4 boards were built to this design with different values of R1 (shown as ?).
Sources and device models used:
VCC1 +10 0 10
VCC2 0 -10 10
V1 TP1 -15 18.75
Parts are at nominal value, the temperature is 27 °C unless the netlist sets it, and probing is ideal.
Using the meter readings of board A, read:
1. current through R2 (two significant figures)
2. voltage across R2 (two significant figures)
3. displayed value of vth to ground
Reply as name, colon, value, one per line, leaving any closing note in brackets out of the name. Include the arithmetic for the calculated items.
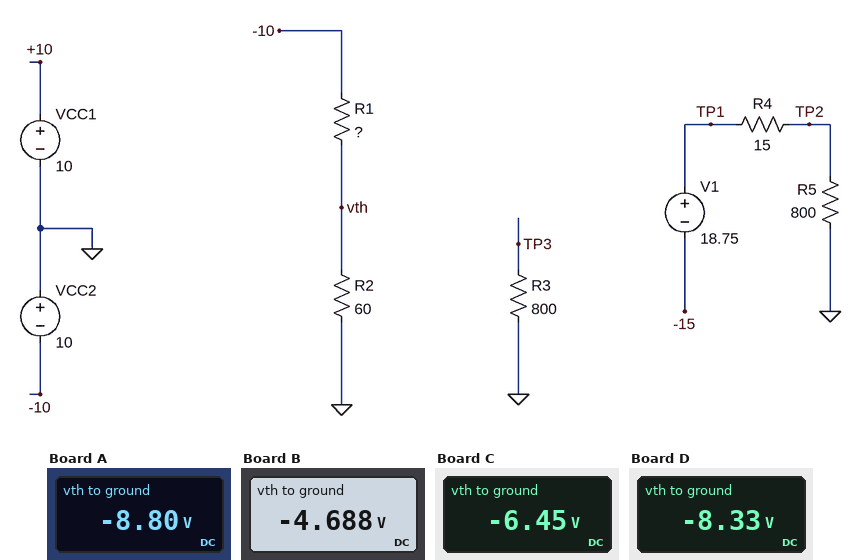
current through R2: (0 V - (-8.8 V)) / 60 Ω = 150 mA
voltage across R2: 0 V - (-8.8 V) = 8.8 V
displayed value of vth to ground: -8.80 V
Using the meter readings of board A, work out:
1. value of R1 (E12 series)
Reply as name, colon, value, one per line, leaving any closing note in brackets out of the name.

value of R1: 8.2 Ω
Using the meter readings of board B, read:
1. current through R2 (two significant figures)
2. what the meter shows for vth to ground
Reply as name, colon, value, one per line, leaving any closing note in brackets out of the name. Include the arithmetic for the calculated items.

current through R2: (0 V - (-4.688 V)) / 60 Ω = 78 mA
what the meter shows for vth to ground: -4.688 V
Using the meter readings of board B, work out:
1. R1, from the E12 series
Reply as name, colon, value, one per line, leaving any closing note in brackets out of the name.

R1, from the E12 series: 68 Ω
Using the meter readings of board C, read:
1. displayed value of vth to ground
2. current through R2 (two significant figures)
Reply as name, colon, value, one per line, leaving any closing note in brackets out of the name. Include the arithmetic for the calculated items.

displayed value of vth to ground: -6.45 V
current through R2: (0 V - (-6.45 V)) / 60 Ω = 110 mA
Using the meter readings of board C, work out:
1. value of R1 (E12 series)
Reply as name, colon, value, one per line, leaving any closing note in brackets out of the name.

value of R1: 33 Ω
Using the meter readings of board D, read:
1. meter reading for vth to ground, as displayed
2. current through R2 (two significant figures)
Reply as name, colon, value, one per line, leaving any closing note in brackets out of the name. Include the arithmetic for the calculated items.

meter reading for vth to ground, as displayed: -8.33 V
current through R2: (0 V - (-8.33 V)) / 60 Ω = 140 mA
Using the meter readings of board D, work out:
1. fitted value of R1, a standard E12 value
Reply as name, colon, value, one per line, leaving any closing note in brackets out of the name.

fitted value of R1, a standard E12 value: 12 Ω
